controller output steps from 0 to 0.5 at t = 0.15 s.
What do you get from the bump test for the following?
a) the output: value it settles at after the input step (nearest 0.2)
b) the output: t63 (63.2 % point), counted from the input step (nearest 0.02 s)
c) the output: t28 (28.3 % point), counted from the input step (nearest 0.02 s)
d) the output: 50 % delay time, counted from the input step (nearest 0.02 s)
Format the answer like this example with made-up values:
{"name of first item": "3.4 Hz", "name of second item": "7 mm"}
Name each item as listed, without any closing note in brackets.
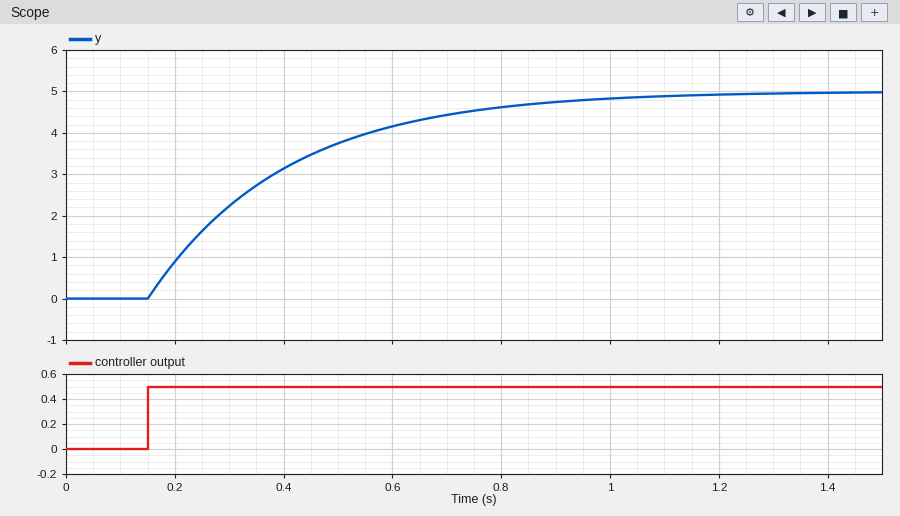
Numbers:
{"the output: value it settles at after the input step": "5.0", "the output: t63 (63.2 % point), counted from the input step": "0.26 s", "the output: t28 (28.3 % point), counted from the input step": "0.08 s", "the output: 50 % delay time, counted from the input step": "0.18 s"}
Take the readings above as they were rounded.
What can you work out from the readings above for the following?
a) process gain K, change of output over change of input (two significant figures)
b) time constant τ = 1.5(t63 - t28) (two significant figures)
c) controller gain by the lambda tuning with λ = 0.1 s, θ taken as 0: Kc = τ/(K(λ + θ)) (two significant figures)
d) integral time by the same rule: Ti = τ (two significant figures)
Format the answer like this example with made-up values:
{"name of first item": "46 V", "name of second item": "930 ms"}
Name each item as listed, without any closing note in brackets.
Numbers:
{"process gain K, change of output over change of input": "10", "time constant τ = 1.5(t63 - t28)": "0.27 s", "controller gain by the lambda tuning with λ = 0.1 s, θ taken as 0: Kc = τ/(K(λ + θ))": "0.27", "integral time by the same rule: Ti = τ": "0.27 s"}
